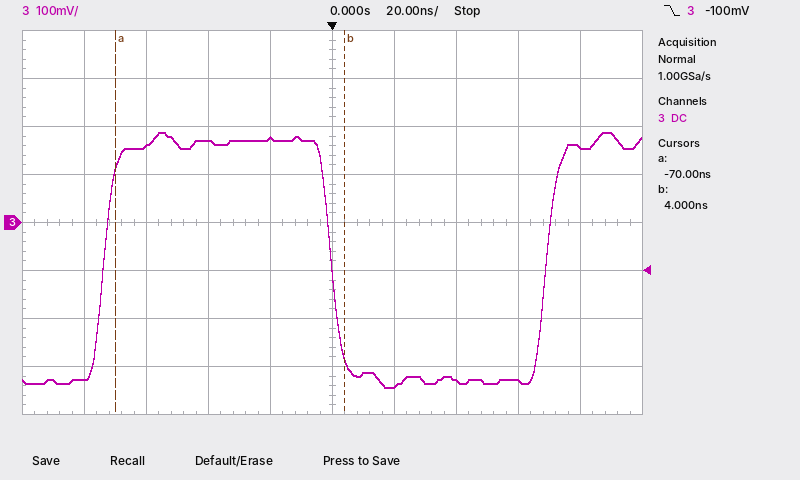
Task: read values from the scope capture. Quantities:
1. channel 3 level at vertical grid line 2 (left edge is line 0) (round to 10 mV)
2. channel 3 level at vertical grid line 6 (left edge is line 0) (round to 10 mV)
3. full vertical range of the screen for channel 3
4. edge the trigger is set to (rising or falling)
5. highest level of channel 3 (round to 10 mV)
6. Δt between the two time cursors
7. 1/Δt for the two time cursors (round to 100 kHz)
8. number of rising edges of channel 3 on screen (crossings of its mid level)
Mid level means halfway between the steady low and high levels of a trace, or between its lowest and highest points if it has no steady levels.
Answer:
160 mV
-340 mV
800 mV
falling
190 mV
74 ns
13.5 MHz
2
